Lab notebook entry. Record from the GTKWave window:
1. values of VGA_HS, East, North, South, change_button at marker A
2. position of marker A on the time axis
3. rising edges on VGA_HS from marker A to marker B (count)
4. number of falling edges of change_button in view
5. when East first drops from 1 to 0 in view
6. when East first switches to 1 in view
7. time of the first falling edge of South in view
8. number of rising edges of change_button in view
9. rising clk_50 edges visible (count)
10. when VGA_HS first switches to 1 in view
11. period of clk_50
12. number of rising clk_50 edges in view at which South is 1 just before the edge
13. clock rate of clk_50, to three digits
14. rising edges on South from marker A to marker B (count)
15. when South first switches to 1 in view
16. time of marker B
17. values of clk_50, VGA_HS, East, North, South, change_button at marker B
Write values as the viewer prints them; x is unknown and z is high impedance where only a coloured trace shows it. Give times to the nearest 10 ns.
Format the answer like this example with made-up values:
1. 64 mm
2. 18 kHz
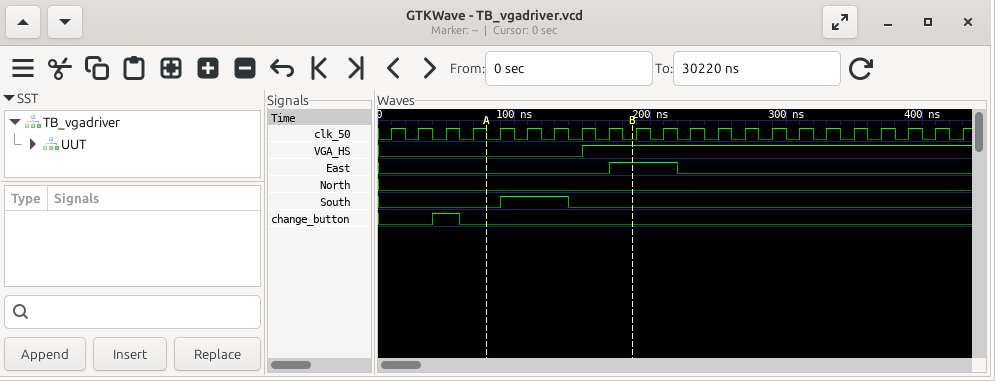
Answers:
1. VGA_HS=0, East=0, North=0, South=0, change_button=0
2. 80 ns
3. 1
4. 1
5. 220 ns
6. 170 ns
7. 140 ns
8. 1
9. 22
10. 150 ns
11. 20 ns
12. 2
13. 50.0 MHz
14. 1
15. 90 ns
16. 190 ns
17. clk_50=0, VGA_HS=1, East=1, North=0, South=0, change_button=0
